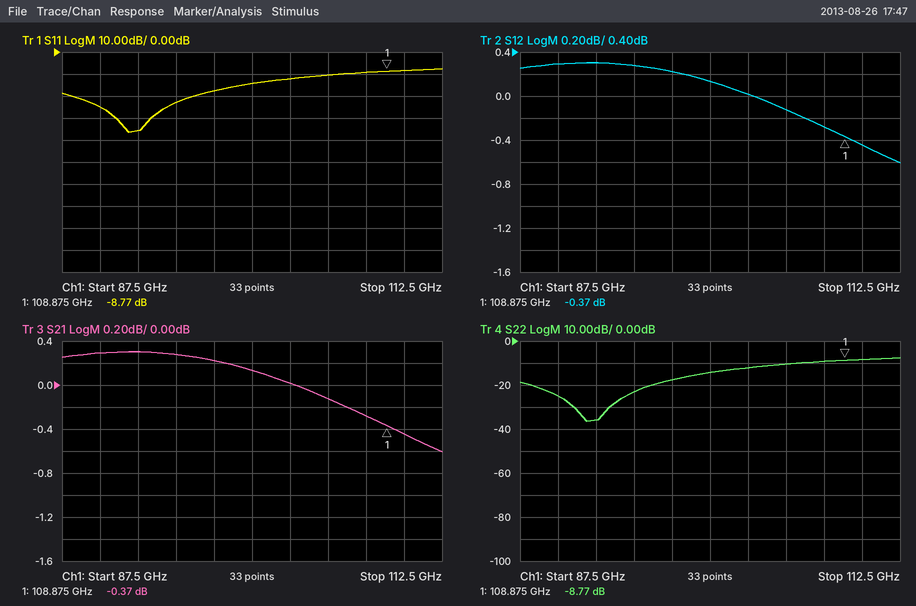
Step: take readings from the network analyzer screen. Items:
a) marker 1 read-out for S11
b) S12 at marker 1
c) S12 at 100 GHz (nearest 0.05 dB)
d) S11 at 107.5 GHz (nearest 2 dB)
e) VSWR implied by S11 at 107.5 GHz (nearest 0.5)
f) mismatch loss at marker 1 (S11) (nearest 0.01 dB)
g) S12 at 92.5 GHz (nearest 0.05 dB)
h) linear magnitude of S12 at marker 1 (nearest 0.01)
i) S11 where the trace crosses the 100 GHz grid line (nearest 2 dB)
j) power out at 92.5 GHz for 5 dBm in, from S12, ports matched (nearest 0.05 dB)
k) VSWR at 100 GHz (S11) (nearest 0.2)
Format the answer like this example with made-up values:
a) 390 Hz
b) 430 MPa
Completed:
a) -8.77 dB
b) -0.37 dB
c) 0.15 dB
d) -10 dB
e) 2.0
f) 0.62 dB
g) 0.30 dB
h) 0.96
i) -14 dB
j) 5.30 dBm
k) 1.4
